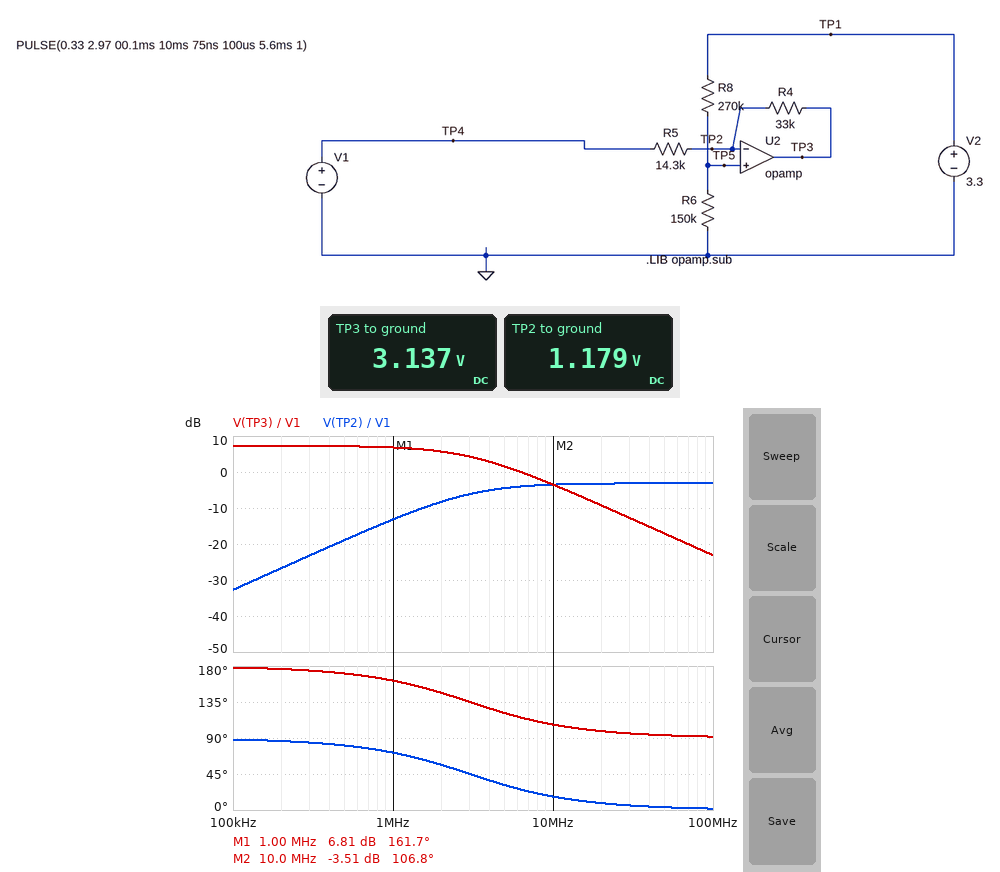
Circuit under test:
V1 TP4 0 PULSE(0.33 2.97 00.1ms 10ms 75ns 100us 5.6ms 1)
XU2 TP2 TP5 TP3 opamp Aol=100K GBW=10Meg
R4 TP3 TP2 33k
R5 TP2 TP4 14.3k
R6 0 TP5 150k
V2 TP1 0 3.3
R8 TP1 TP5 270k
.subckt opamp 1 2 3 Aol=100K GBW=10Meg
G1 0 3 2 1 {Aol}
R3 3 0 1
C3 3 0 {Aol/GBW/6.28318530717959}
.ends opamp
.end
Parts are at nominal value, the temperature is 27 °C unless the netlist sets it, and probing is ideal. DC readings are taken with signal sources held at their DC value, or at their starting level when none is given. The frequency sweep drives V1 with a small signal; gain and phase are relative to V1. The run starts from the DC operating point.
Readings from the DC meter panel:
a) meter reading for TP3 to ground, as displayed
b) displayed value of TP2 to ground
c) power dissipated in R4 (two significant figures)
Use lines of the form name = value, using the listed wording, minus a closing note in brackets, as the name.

meter reading for TP3 to ground, as displayed = 3.137 V
displayed value of TP2 to ground = 1.179 V
power dissipated in R4 = 120 µW
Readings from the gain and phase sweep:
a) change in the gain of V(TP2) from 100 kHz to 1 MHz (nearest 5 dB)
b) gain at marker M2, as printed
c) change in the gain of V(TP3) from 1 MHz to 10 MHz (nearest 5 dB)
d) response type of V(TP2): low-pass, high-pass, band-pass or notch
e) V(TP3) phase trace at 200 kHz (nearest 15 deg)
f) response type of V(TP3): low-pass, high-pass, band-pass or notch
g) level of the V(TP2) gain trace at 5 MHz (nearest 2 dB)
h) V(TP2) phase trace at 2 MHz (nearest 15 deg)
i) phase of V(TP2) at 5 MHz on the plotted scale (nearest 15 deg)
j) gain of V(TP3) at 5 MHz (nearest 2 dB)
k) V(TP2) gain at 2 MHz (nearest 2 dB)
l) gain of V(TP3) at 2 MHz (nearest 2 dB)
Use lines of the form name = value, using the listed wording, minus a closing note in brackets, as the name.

change in the gain of V(TP2) from 100 kHz to 1 MHz = 20 dB
gain at marker M2, as printed = -3.51 dB
change in the gain of V(TP3) from 1 MHz to 10 MHz = -10 dB
response type of V(TP2): low-pass, high-pass, band-pass or notch = high-pass
V(TP3) phase trace at 200 kHz = 180 deg
response type of V(TP3): low-pass, high-pass, band-pass or notch = low-pass
level of the V(TP2) gain trace at 5 MHz = -4 dB
V(TP2) phase trace at 2 MHz = 60 deg
phase of V(TP2) at 5 MHz on the plotted scale = 30 deg
gain of V(TP3) at 5 MHz = 2 dB
V(TP2) gain at 2 MHz = -8 dB
gain of V(TP3) at 2 MHz = 6 dB
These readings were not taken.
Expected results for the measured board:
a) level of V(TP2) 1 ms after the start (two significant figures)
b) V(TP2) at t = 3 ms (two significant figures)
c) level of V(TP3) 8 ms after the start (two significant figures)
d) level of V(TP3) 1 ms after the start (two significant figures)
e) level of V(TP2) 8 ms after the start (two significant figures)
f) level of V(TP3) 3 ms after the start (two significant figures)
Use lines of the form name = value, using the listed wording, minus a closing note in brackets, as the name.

level of V(TP2) 1 ms after the start = 1.2 V
V(TP2) at t = 3 ms = 1.2 V
level of V(TP3) 8 ms after the start = 3.1 V
level of V(TP3) 1 ms after the start = 2.6 V
level of V(TP2) 8 ms after the start = 1.2 V
level of V(TP3) 3 ms after the start = 1.4 V
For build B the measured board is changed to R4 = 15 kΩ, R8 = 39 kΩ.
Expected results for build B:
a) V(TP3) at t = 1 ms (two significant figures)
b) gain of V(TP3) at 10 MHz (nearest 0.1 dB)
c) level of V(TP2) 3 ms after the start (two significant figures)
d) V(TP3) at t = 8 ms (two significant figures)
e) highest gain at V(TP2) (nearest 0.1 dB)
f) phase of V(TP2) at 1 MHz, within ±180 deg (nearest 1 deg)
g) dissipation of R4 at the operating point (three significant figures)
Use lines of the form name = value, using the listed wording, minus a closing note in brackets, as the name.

V(TP3) at t = 1 ms = 4.8 V
gain of V(TP3) at 10 MHz = -6.7 dB
level of V(TP2) 3 ms after the start = 2.6 V
V(TP3) at t = 8 ms = 5.0 V
highest gain at V(TP2) = -5.8 dB
phase of V(TP2) at 1 MHz, within ±180 deg = 78 deg
dissipation of R4 at the operating point = 384 µW
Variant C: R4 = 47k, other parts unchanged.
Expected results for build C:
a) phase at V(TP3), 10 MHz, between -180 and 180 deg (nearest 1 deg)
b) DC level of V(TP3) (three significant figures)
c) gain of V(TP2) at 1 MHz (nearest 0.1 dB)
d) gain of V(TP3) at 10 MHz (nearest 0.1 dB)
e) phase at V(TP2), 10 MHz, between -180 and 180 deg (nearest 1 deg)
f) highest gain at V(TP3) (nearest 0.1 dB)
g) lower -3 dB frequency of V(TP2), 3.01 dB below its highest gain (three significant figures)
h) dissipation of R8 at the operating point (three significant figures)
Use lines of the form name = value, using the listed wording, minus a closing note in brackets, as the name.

phase at V(TP3), 10 MHz, between -180 and 180 deg = 103 deg
DC level of V(TP3) = 3.97 V
gain of V(TP2) at 1 MHz = -10.4 dB
gain of V(TP3) at 10 MHz = -2.5 dB
phase at V(TP2), 10 MHz, between -180 and 180 deg = 13 deg
highest gain at V(TP3) = 10.3 dB
lower -3 dB frequency of V(TP2), 3.01 dB below its highest gain = 2.33 MHz
dissipation of R8 at the operating point = 16.7 µW
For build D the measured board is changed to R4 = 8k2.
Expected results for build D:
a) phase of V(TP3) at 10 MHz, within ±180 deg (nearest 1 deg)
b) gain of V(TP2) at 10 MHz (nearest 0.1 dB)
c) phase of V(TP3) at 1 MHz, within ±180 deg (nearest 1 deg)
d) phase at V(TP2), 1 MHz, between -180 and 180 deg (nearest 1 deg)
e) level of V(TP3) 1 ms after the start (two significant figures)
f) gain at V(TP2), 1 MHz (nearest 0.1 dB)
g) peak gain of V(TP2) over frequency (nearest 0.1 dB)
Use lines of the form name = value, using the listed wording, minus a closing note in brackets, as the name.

phase of V(TP3) at 10 MHz, within ±180 deg = 122 deg
gain of V(TP2) at 10 MHz = -10.2 dB
phase of V(TP3) at 1 MHz, within ±180 deg = 171 deg
phase at V(TP2), 1 MHz, between -180 and 180 deg = 81 deg
level of V(TP3) 1 ms after the start = 1.5 V
gain at V(TP2), 1 MHz = -24.9 dB
peak gain of V(TP2) over frequency = -8.8 dB
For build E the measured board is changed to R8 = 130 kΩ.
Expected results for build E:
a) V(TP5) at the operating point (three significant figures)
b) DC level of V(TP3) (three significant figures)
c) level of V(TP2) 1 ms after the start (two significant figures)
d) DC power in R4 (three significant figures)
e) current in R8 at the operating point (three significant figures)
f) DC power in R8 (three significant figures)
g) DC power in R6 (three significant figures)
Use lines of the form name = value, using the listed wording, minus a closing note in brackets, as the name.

V(TP5) at the operating point = 1.77 V
DC level of V(TP3) = 5.09 V
level of V(TP2) 1 ms after the start = 1.8 V
DC power in R4 = 334 µW
current in R8 at the operating point = 11.8 µA
DC power in R8 = 18.1 µW
DC power in R6 = 20.8 µW
